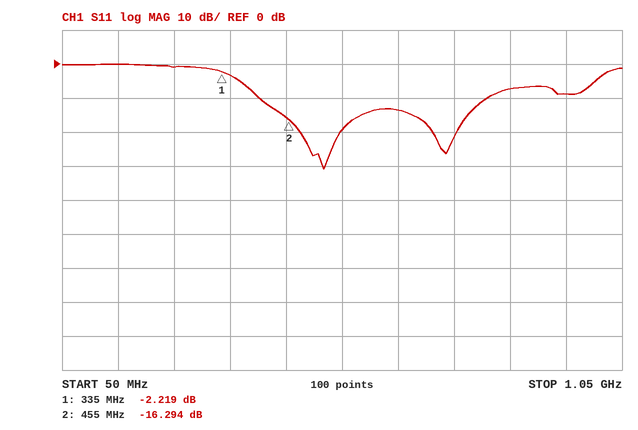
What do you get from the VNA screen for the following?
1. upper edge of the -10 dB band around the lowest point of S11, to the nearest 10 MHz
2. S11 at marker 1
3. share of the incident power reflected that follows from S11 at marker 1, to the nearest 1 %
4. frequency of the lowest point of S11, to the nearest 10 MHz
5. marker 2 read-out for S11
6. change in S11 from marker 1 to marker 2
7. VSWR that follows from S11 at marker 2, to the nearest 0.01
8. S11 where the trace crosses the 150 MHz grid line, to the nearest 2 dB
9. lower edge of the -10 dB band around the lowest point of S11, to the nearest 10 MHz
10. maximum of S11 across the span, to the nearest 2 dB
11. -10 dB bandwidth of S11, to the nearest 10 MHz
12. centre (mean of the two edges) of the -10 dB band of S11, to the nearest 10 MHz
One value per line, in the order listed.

810 MHz
-2.219 dB
60 %
520 MHz
-16.294 dB
-14.075 dB
1.36
0 dB
400 MHz
0 dB
410 MHz
610 MHz
